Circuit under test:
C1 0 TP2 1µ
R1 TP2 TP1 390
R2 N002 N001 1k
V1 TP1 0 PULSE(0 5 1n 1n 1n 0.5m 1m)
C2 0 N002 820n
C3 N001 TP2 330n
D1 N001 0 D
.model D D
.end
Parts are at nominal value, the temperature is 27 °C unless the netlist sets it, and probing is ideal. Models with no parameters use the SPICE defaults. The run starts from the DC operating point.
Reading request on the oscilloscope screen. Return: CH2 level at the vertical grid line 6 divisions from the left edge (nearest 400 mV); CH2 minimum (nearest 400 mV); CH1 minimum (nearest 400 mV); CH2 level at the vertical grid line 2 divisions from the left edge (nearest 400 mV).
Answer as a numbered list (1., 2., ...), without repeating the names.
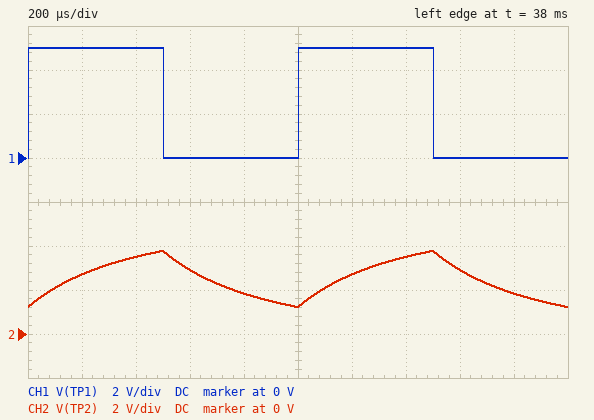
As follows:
1. 2.8 V
2. 1.2 V
3. 0 V
4. 3.6 V
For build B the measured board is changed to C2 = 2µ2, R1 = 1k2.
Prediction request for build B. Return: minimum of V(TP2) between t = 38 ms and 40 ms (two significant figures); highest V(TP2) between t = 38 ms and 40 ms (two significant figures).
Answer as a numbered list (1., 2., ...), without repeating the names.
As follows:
1. 2.0 V
2. 3.0 V
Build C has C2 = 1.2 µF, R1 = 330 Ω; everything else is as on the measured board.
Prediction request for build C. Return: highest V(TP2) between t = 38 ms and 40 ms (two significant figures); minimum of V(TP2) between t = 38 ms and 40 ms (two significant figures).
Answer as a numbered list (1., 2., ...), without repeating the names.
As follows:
1. 3.9 V
2. 1.1 V
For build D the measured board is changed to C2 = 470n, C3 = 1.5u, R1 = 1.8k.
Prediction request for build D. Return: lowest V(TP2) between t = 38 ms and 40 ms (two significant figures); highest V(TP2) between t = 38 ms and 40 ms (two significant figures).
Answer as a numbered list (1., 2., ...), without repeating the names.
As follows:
1. 2.2 V
2. 2.8 V
